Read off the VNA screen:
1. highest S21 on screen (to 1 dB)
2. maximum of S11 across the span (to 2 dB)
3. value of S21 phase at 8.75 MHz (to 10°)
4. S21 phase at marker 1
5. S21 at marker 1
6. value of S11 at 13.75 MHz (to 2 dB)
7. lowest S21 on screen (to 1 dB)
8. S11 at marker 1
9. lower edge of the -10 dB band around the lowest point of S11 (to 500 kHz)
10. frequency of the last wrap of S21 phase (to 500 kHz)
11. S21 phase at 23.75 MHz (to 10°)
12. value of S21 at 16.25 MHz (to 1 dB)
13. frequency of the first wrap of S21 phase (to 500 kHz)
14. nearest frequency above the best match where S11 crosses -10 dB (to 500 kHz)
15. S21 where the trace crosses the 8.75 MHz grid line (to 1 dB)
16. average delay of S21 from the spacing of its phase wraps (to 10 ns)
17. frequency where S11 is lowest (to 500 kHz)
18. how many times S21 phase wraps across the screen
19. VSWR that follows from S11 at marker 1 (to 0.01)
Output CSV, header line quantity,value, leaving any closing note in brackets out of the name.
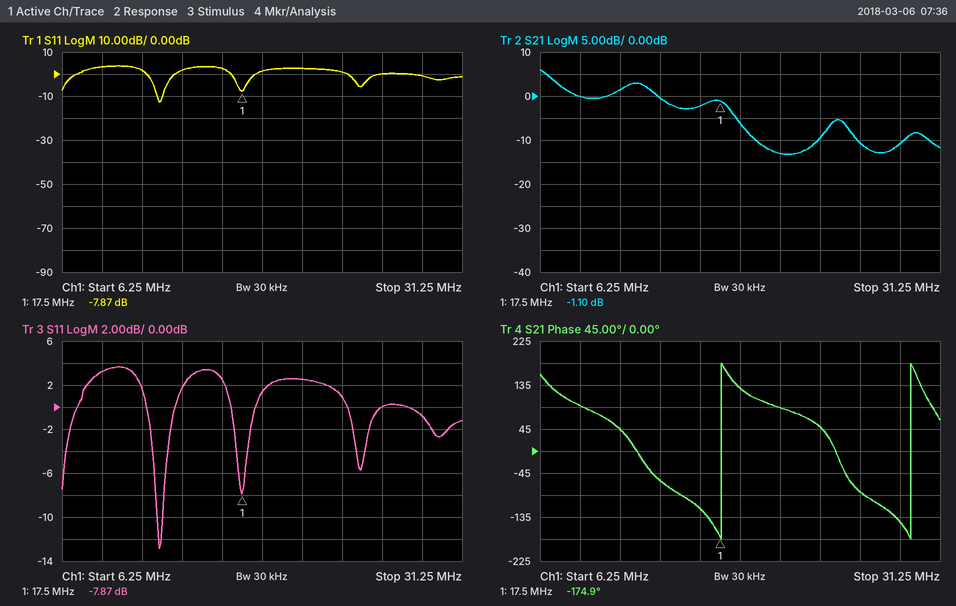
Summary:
quantity,value
highest S21 on screen,6 dB
maximum of S11 across the span,4 dB
value of S21 phase at 8.75 MHz,90°
S21 phase at marker 1,-174.9°
S21 at marker 1,-1.10 dB
value of S11 at 13.75 MHz,2 dB
lowest S21 on screen,-13 dB
S11 at marker 1,-7.87 dB
lower edge of the -10 dB band around the lowest point of S11,12.0 MHz
frequency of the last wrap of S21 phase,29.5 MHz
S21 phase at 23.75 MHz,50°
value of S21 at 16.25 MHz,-2 dB
frequency of the first wrap of S21 phase,17.5 MHz
nearest frequency above the best match where S11 crosses -10 dB,12.5 MHz
S21 where the trace crosses the 8.75 MHz grid line,0 dB
average delay of S21 from the spacing of its phase wraps,80 ns
frequency where S11 is lowest,12.5 MHz
how many times S21 phase wraps across the screen,2
VSWR that follows from S11 at marker 1,2.36
